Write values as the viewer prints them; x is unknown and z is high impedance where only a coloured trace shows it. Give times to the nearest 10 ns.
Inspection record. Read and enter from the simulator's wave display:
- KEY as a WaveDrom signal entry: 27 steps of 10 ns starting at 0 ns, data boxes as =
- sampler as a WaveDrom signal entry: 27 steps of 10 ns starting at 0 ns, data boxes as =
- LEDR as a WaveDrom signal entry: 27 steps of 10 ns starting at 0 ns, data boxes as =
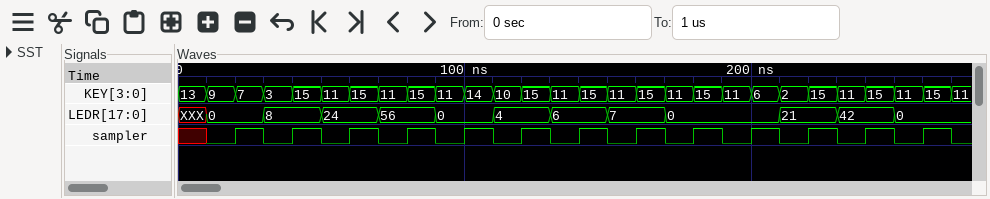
{name: 'KEY', wave: '===========================', data: '13 9 7 3 15 11 15 11 15 11 14 10 15 11 15 11 15 11 15 11 6 2 15 11 15 11 15'}
{name: 'sampler', wave: 'x01010101010101010101010101'}
{name: 'LEDR', wave: '==.=.=.=.=.=.=.=.=...=.=.=.', data: 'XXX 0 8 24 56 0 4 6 7 0 21 42 0'}
